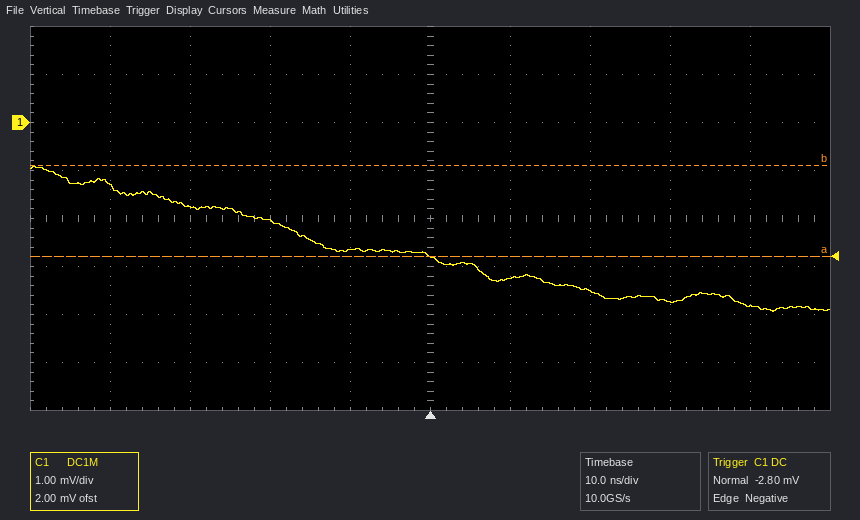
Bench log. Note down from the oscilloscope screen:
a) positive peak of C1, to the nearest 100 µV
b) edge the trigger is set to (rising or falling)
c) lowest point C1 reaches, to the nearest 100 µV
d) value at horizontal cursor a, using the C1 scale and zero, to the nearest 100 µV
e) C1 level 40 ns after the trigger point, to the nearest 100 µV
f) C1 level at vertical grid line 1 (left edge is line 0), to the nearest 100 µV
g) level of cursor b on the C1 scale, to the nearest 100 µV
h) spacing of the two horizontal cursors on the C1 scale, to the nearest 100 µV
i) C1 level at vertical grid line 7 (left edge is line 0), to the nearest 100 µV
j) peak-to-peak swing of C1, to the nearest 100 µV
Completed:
-900 µV
falling
-3.9 mV
-2.8 mV
-3.8 mV
-1.3 mV
-900 µV
1.9 mV
-3.5 mV
3.0 mV
